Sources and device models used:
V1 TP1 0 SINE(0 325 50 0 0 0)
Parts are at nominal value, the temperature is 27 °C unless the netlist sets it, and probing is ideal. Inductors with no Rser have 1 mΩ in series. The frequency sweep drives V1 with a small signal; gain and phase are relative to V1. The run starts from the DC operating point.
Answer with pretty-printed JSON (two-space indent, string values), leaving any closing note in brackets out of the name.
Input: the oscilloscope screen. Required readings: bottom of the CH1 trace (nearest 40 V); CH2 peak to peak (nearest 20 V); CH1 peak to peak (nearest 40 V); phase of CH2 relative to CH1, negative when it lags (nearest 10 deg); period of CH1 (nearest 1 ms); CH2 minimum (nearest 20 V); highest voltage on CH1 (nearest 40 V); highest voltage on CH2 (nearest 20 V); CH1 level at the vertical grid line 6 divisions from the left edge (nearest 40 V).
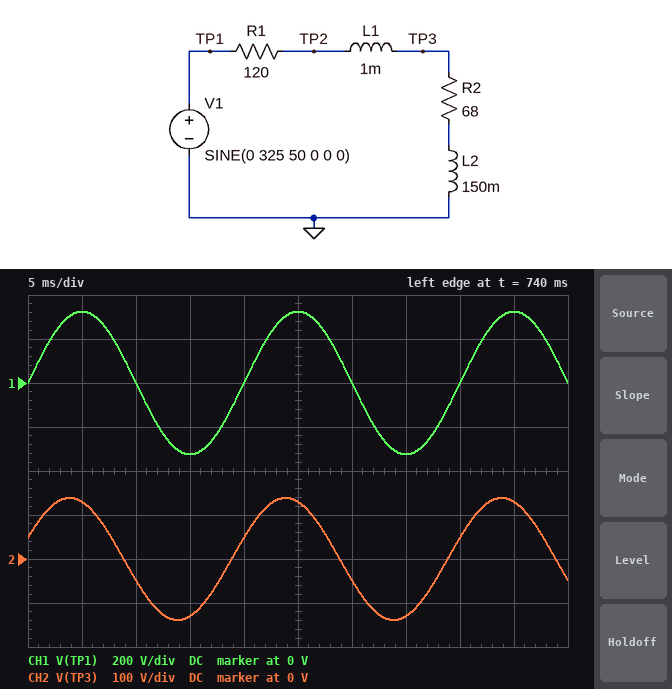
{
  "bottom of the CH1 trace": "-320 V",
  "CH2 peak to peak": "280 V",
  "CH1 peak to peak": "640 V",
  "phase of CH2 relative to CH1, negative when it lags": "20 deg",
  "period of CH1": "20 ms",
  "CH2 minimum": "-140 V",
  "highest voltage on CH1": "320 V",
  "highest voltage on CH2": "140 V",
  "CH1 level at the vertical grid line 6 divisions from the left edge": "0 V"
}
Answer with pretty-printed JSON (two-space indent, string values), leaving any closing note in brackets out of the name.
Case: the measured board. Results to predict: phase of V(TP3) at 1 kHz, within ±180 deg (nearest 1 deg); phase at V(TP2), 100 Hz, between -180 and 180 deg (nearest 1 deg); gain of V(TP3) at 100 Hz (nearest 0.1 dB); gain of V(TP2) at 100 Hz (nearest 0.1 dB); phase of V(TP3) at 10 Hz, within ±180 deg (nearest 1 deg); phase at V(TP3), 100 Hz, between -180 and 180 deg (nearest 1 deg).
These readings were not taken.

{
  "phase of V(TP3) at 1 kHz, within ±180 deg": "7 deg",
  "phase at V(TP2), 100 Hz, between -180 and 180 deg": "28 deg",
  "gain of V(TP3) at 100 Hz": "-5.2 dB",
  "gain of V(TP2) at 100 Hz": "-5.1 dB",
  "phase of V(TP3) at 10 Hz, within ±180 deg": "5 deg",
  "phase at V(TP3), 100 Hz, between -180 and 180 deg": "27 deg"
}
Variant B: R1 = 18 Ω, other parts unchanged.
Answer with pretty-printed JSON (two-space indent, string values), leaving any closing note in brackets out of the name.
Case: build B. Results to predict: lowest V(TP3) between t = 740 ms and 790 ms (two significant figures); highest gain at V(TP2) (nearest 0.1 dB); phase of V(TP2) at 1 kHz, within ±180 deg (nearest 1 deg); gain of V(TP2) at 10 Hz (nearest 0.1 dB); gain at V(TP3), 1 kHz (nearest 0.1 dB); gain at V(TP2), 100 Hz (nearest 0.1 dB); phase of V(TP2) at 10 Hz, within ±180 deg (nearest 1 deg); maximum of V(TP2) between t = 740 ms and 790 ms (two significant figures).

{
  "lowest V(TP3) between t = 740 ms and 790 ms": "-270 V",
  "highest gain at V(TP2)": "0 dB",
  "phase of V(TP2) at 1 kHz, within ±180 deg": "1 deg",
  "gain of V(TP2) at 10 Hz": "-2.0 dB",
  "gain at V(TP3), 1 kHz": "-0.1 dB",
  "gain at V(TP2), 100 Hz": "-0.8 dB",
  "phase of V(TP2) at 10 Hz, within ±180 deg": "2 deg",
  "maximum of V(TP2) between t = 740 ms and 790 ms": "270 V"
}
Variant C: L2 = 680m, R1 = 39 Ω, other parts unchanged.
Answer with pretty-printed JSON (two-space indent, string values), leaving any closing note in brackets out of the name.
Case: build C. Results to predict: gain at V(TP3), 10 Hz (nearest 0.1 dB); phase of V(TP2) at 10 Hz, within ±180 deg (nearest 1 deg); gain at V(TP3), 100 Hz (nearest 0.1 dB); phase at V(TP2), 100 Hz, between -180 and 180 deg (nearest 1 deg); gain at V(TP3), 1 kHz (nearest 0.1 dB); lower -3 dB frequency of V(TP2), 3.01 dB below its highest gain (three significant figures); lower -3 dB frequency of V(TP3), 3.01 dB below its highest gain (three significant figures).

{
  "gain at V(TP3), 10 Hz": "-3.1 dB",
  "phase of V(TP2) at 10 Hz, within ±180 deg": "10 deg",
  "gain at V(TP3), 100 Hz": "-0.2 dB",
  "phase at V(TP2), 100 Hz, between -180 and 180 deg": "5 deg",
  "gain at V(TP3), 1 kHz": "0 dB",
  "lower -3 dB frequency of V(TP2), 3.01 dB below its highest gain": "11.0 Hz",
  "lower -3 dB frequency of V(TP3), 3.01 dB below its highest gain": "10.9 Hz"
}
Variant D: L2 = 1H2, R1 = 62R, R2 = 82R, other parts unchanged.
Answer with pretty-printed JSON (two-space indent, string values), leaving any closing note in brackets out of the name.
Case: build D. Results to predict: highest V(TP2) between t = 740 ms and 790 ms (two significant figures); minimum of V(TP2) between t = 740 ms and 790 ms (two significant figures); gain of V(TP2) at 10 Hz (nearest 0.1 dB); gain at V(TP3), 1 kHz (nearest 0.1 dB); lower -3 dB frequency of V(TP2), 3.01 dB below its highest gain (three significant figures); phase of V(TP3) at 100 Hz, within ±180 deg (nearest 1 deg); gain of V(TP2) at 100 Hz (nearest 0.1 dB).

{
  "highest V(TP2) between t = 740 ms and 790 ms": "310 V",
  "minimum of V(TP2) between t = 740 ms and 790 ms": "-310 V",
  "gain of V(TP2) at 10 Hz": "-3.3 dB",
  "gain at V(TP3), 1 kHz": "0 dB",
  "lower -3 dB frequency of V(TP2), 3.01 dB below its highest gain": "11.3 Hz",
  "phase of V(TP3) at 100 Hz, within ±180 deg": "5 deg",
  "gain of V(TP2) at 100 Hz": "-0.1 dB"
}
